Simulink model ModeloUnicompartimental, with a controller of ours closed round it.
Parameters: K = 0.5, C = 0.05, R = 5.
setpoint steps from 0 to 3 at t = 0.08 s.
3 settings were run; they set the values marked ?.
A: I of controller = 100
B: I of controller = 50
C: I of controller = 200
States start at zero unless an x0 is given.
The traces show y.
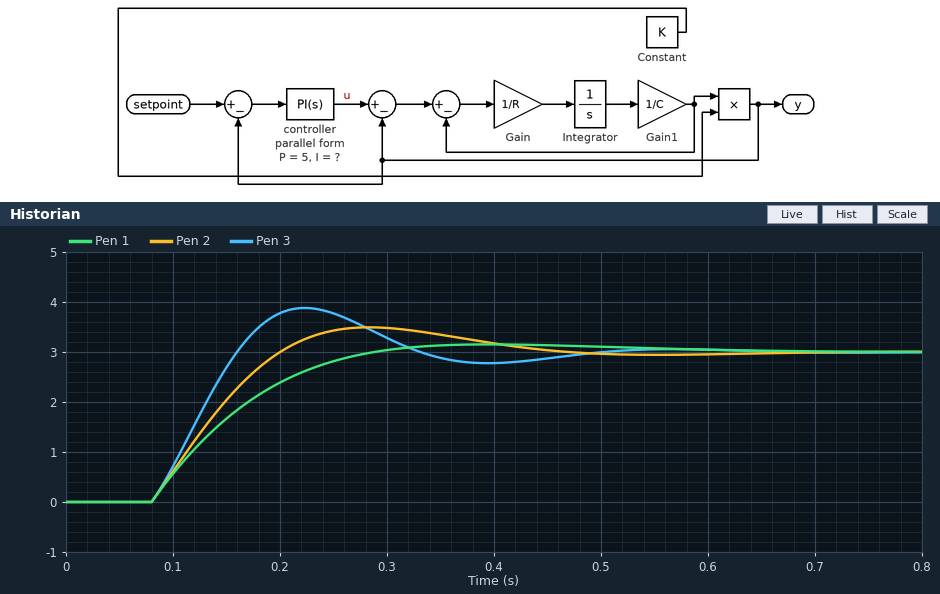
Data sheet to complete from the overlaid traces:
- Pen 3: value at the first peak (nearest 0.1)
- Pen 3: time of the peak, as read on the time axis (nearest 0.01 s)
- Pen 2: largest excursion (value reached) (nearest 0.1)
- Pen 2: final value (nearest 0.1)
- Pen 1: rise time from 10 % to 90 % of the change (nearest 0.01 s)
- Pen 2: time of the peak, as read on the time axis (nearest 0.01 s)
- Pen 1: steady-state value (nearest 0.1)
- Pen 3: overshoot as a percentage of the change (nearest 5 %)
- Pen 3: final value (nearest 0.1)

3.9
0.22 s
3.5
3.0
0.14 s
0.28 s
3.0
30 %
3.0
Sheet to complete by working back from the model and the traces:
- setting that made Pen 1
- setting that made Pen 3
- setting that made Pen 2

B
C
A
